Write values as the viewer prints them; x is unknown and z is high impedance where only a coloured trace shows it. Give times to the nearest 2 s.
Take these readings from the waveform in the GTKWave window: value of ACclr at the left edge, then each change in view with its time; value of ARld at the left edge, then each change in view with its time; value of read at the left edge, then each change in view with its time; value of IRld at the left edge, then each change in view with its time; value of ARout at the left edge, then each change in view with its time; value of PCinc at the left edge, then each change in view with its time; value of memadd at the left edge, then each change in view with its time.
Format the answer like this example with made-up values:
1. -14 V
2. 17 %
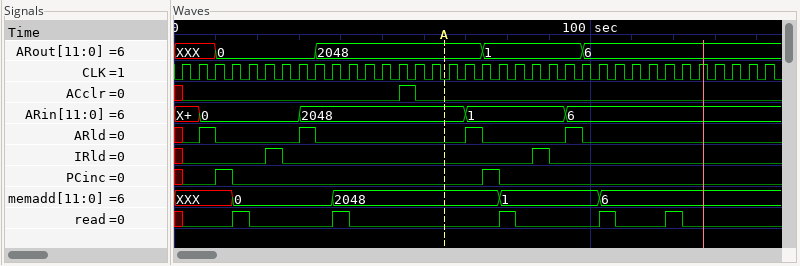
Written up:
1. x, 0 at 2 s, 1 at 54 s, 0 at 58 s
2. x, 0 at 2 s, 1 at 6 s, 0 at 10 s, 1 at 30 s, 0 at 34 s, 1 at 70 s, 0 at 74 s, 1 at 94 s, 0 at 98 s
3. x, 0 at 2 s, 1 at 14 s, 0 at 18 s, 1 at 38 s, 0 at 42 s, 1 at 78 s, 0 at 82 s, 1 at 102 s, 0 at 106 s, 1 at 118 s, 0 at 122 s
4. x, 0 at 2 s, 1 at 22 s, 0 at 26 s, 1 at 86 s, 0 at 90 s
5. XXX, 0 at 10 s, 2048 at 34 s, 1 at 74 s, 6 at 98 s
6. x, 0 at 2 s, 1 at 10 s, 0 at 14 s, 1 at 74 s, 0 at 78 s
7. XXX, 0 at 14 s, 2048 at 38 s, 1 at 78 s, 6 at 102 s
